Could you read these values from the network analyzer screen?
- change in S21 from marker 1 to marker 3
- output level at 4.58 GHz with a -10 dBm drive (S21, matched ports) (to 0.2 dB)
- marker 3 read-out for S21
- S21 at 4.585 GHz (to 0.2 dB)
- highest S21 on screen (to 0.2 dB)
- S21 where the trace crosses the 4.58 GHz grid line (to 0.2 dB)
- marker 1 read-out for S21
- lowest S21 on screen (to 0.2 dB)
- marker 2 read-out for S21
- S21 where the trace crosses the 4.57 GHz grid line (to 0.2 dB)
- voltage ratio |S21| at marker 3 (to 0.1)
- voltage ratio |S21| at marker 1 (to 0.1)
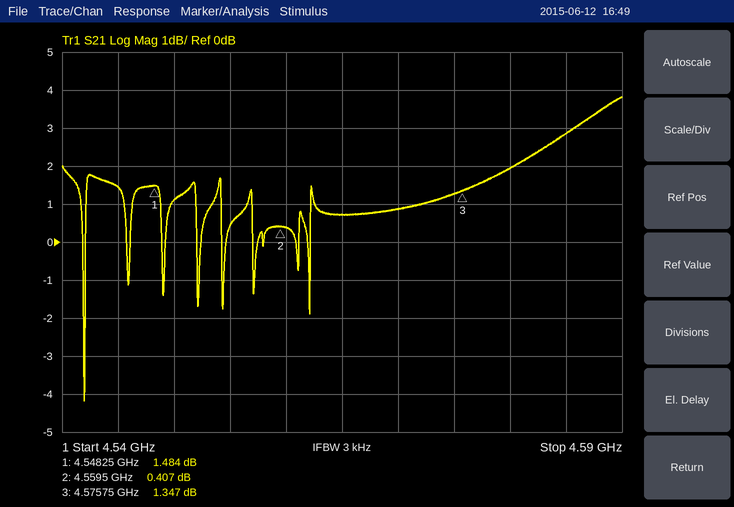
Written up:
-0.137 dB
-8.0 dBm
1.347 dB
2.8 dB
3.8 dB
2.0 dB
1.484 dB
-4.2 dB
0.407 dB
0.8 dB
1.2
1.2
